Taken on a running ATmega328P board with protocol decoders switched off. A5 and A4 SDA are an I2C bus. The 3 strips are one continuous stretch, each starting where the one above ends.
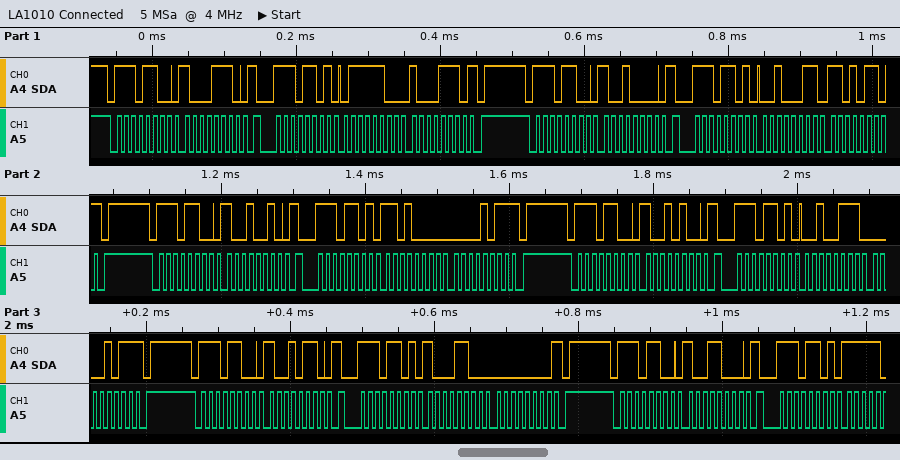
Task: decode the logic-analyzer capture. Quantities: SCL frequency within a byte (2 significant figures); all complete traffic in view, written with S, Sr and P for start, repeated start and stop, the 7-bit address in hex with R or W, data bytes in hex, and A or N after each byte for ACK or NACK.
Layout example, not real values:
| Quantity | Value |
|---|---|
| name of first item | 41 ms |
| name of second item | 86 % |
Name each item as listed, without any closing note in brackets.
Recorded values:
| Quantity | Value |
|---|---|
| SCL frequency within a byte | 100 kHz |
| all complete traffic in view, written with S, Sr and P for start, repeated start and stop, the 7-bit address in hex with R or W, data bytes in hex, and A or N after each byte for ACK or NACK | S 76W A 8E A Sr 76R A 7C A 8E N P S 76W A 90 A Sr 76R A 23 A D6 N P S 76W A 92 A Sr 76R A D0 A 0B N P S 76W A 94 A Sr 76R A 27 A 0B N P S 76W A 96 A Sr 76R A 8C A 00 N P S 76W A 98 A Sr 76R A |
